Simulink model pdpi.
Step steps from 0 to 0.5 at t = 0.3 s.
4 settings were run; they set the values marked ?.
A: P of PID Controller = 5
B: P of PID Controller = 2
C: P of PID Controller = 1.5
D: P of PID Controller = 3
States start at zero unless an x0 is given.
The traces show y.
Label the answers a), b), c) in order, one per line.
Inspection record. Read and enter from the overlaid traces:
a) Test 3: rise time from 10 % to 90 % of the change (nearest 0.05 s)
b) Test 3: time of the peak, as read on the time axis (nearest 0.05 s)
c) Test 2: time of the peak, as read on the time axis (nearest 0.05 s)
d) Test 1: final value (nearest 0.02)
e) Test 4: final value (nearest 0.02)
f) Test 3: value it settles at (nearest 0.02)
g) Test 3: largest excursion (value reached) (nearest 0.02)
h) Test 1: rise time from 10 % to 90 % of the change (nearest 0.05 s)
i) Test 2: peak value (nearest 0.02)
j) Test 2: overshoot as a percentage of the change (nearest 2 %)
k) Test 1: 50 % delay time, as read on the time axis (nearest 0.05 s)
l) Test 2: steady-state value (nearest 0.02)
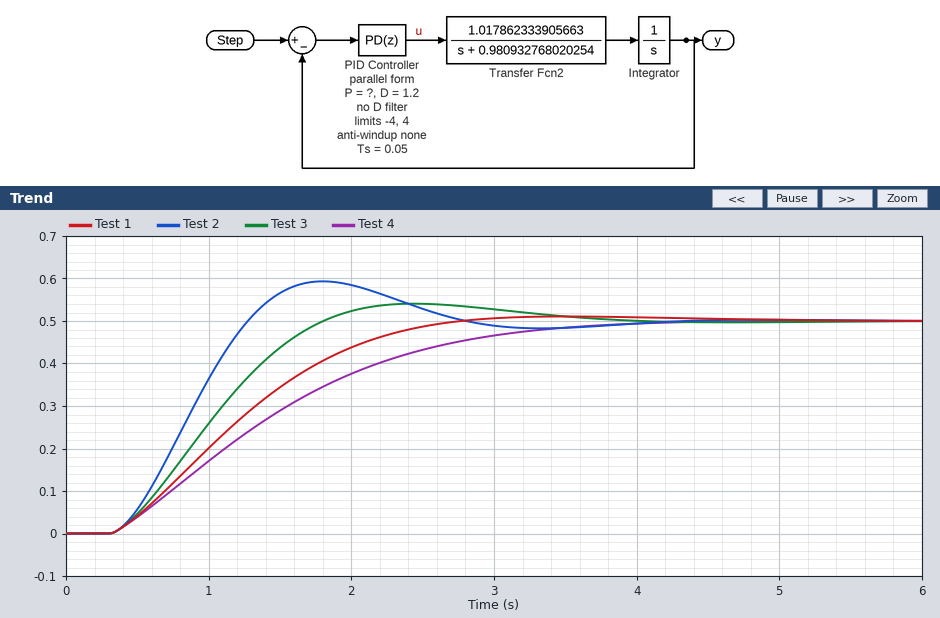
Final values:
a) 1.05 s
b) 2.45 s
c) 1.80 s
d) 0.50
e) 0.50
f) 0.50
g) 0.54
h) 1.55 s
i) 0.60
j) 18 %
k) 1.15 s
l) 0.50
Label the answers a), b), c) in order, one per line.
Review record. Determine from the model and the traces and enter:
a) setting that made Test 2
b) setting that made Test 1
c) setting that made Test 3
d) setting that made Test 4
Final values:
a) A
b) B
c) D
d) C
